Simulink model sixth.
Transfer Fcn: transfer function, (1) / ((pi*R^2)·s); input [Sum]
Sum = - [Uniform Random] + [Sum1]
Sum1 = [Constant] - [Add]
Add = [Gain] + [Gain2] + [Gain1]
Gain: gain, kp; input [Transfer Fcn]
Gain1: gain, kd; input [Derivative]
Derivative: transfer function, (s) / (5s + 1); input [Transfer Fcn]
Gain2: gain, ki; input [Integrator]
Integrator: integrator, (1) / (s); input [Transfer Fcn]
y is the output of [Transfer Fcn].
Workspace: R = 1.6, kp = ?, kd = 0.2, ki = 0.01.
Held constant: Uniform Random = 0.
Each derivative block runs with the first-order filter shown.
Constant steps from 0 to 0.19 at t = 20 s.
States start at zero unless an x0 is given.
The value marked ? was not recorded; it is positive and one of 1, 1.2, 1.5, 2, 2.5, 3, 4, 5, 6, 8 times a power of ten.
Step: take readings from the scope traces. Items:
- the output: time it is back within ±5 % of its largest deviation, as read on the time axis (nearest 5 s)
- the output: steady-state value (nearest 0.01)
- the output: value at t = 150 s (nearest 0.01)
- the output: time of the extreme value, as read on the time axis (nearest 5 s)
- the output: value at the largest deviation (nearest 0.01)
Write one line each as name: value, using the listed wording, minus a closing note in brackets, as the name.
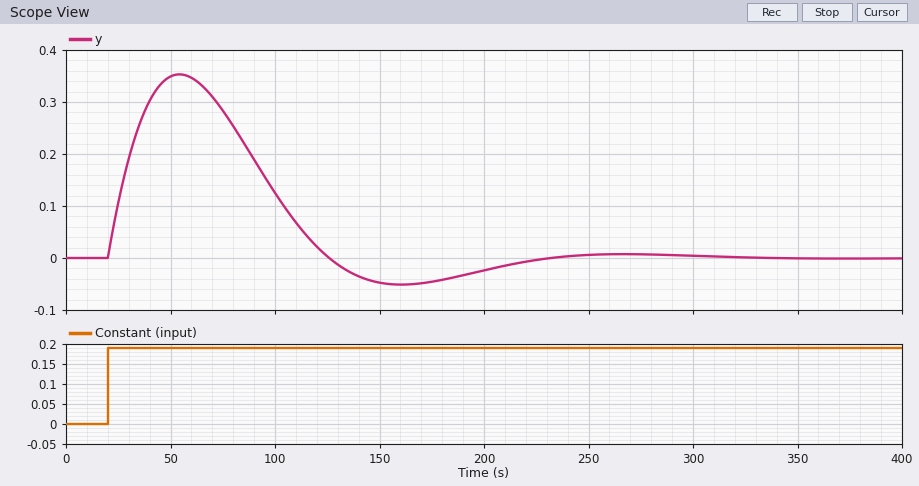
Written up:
the output: time it is back within ±5 % of its largest deviation, as read on the time axis: 205 s
the output: steady-state value: 0.00
the output: value at t = 150 s: -0.05
the output: time of the extreme value, as read on the time axis: 55 s
the output: value at the largest deviation: 0.35
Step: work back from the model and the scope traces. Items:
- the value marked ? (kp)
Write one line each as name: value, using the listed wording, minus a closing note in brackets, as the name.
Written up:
the value marked ?: 0.3
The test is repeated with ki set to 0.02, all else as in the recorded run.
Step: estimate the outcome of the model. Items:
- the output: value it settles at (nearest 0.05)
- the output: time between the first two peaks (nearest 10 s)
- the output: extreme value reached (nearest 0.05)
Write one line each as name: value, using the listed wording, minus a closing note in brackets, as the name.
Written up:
the output: value it settles at: 0.00
the output: time between the first two peaks: 140 s
the output: extreme value reached: 0.30
